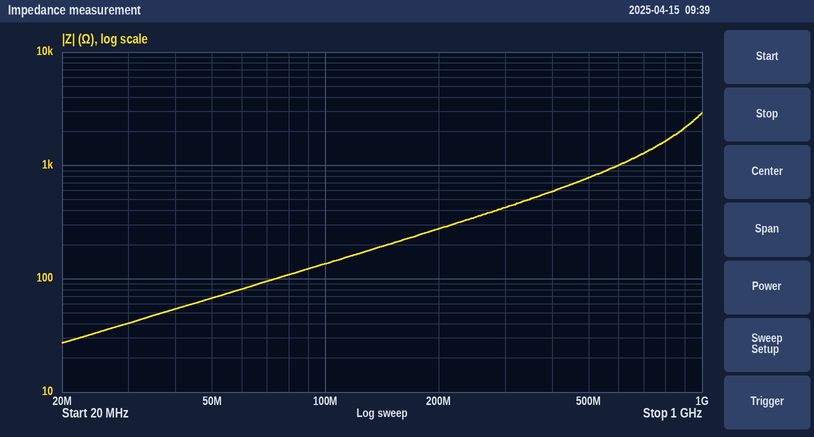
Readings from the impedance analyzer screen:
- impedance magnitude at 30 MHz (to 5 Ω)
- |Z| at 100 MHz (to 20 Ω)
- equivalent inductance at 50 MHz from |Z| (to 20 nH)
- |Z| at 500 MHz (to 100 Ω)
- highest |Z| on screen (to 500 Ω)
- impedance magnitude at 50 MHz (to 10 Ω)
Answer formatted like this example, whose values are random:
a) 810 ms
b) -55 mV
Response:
a) 40 Ω
b) 140 Ω
c) 220 nH
d) 800 Ω
e) 3.0 kΩ
f) 70 Ω
